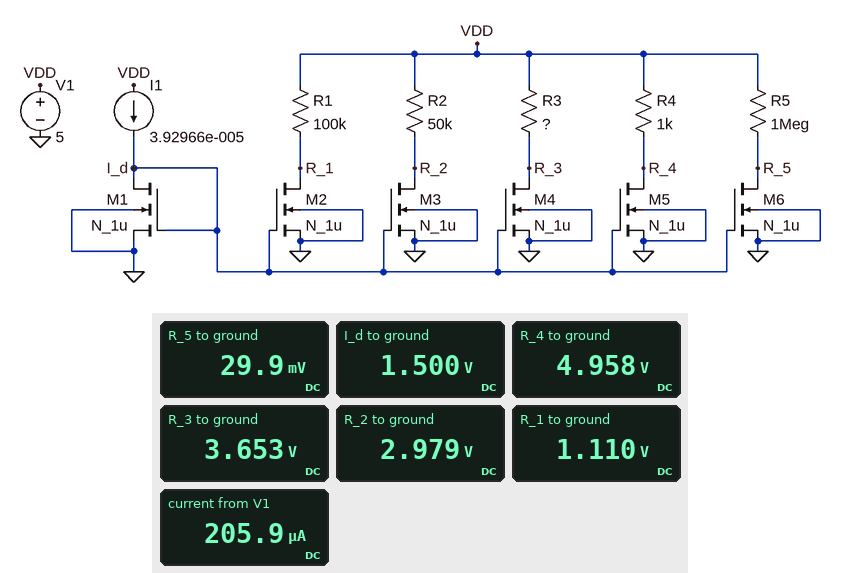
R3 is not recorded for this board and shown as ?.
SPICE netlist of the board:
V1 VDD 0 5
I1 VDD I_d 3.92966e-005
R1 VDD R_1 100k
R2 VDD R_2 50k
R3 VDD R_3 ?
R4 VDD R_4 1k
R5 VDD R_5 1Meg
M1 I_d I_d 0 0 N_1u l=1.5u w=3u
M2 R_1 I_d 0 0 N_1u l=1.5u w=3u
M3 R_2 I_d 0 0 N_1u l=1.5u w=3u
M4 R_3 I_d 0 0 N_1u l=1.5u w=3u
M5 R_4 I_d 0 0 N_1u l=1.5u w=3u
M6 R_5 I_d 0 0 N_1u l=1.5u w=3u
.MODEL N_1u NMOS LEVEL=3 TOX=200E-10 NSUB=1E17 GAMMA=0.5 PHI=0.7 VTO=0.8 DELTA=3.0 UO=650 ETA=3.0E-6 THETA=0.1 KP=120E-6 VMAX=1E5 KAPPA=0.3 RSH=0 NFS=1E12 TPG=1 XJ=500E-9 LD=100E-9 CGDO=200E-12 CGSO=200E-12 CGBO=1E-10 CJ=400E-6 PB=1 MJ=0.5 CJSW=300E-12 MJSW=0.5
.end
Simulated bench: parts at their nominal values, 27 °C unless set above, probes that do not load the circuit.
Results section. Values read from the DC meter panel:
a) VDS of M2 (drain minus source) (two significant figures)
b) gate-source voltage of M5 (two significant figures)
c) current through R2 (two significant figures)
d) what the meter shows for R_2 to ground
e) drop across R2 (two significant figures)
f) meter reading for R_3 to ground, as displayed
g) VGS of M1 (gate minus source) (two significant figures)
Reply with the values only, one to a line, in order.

1.1 V
1.5 V
40 µA
2.979 V
2.0 V
3.653 V
1.5 V
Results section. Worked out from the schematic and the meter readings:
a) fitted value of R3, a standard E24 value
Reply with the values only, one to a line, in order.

33 kΩ
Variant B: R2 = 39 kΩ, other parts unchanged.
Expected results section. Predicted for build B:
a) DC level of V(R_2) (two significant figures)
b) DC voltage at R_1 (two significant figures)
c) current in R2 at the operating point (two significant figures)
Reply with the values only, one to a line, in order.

3.4 V
1.1 V
41 µA
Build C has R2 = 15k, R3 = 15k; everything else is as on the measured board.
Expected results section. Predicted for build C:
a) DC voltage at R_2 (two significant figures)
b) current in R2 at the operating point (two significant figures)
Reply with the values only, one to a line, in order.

4.4 V
41 µA
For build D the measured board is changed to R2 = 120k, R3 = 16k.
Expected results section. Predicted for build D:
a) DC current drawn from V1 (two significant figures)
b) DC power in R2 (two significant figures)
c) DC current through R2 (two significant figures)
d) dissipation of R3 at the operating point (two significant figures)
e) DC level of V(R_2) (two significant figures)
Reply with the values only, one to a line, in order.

200 µA
170 µW
38 µA
27 µW
460 mV
